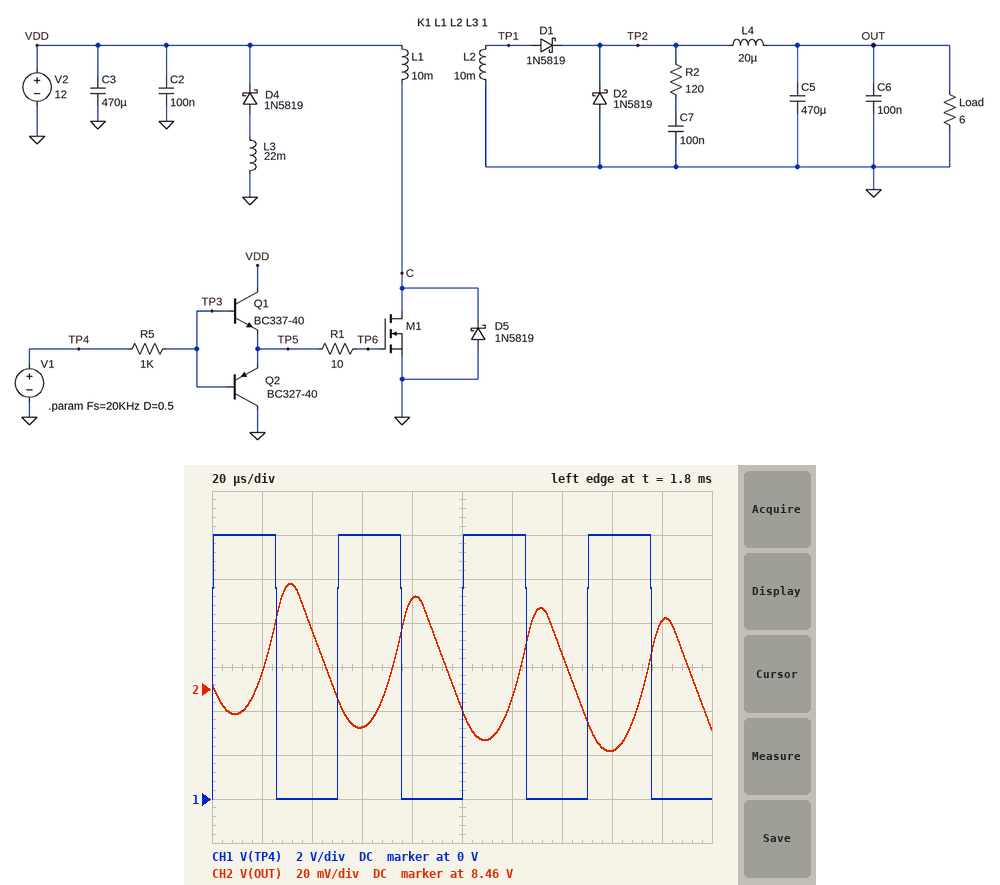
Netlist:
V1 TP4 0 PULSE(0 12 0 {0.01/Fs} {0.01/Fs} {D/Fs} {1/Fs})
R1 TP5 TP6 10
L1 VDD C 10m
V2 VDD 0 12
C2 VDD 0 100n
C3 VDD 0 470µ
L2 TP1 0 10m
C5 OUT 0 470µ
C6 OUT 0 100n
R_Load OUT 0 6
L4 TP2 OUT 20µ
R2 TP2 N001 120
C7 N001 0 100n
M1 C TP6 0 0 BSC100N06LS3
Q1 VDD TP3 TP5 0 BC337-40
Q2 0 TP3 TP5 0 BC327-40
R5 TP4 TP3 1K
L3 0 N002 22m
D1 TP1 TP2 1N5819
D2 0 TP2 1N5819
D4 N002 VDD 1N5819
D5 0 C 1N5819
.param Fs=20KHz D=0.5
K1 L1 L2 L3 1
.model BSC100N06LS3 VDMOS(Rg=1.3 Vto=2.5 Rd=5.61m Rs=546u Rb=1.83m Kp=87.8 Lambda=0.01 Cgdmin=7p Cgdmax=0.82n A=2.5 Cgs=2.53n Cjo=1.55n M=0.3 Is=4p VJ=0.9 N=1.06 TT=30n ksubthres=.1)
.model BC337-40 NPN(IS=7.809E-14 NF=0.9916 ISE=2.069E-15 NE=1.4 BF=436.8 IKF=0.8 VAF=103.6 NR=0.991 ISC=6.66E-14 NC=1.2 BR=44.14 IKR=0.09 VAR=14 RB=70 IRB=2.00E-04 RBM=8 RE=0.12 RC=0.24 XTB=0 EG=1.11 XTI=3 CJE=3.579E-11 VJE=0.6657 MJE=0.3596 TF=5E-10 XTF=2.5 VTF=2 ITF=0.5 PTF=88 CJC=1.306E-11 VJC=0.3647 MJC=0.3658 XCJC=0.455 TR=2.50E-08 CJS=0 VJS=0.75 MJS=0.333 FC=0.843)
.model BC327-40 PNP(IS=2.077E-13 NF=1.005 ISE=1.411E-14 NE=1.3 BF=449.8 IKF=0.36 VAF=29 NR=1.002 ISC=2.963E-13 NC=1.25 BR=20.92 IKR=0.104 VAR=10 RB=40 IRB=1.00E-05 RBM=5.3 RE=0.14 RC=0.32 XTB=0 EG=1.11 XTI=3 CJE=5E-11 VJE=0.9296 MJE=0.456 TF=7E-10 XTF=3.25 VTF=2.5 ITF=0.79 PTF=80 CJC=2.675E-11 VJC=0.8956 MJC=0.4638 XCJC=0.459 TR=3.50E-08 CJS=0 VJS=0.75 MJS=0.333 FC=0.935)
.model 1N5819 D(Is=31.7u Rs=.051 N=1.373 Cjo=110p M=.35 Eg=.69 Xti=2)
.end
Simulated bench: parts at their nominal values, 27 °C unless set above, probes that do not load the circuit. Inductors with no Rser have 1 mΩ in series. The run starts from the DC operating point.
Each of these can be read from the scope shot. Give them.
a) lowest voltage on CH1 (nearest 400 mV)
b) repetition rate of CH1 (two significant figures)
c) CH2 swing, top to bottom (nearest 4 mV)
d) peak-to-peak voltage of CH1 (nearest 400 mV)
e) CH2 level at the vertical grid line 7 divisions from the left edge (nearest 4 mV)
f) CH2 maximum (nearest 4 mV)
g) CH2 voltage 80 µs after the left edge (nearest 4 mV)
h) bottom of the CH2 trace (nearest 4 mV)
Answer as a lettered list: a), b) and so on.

a) 0 V
b) 20 kHz
c) 76 mV
d) 12.0 V
e) 8.476 V
f) 8.508 V
g) 8.500 V
h) 8.432 V
